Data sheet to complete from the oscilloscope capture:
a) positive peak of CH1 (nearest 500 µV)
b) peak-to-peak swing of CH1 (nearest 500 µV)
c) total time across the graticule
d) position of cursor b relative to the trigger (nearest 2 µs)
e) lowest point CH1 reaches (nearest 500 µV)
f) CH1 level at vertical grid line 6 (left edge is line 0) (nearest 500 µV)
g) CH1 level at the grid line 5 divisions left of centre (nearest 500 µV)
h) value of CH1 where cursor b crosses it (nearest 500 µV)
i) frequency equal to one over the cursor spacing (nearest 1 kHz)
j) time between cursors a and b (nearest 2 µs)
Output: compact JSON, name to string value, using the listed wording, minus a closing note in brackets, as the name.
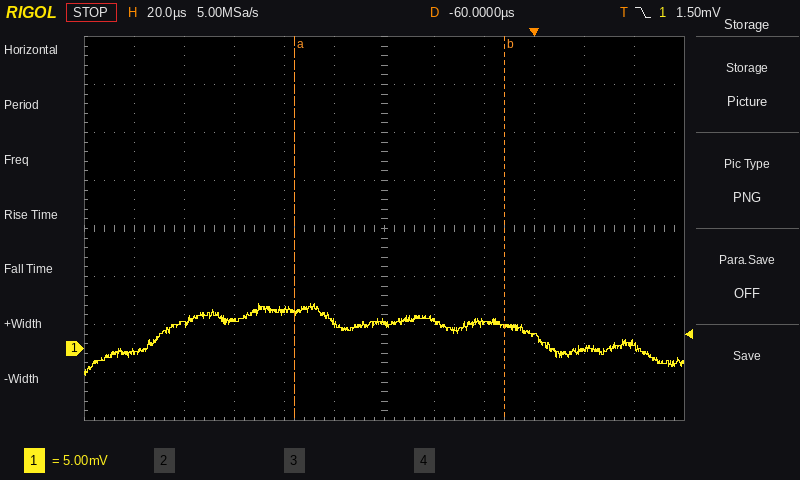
{"positive peak of CH1": "4.5 mV", "peak-to-peak swing of CH1": "7.5 mV", "total time across the graticule": "240 µs", "position of cursor b relative to the trigger": "-12 µs", "lowest point CH1 reaches": "-3.0 mV", "CH1 level at vertical grid line 6 (left edge is line 0)": "2.5 mV", "CH1 level at the grid line 5 divisions left of centre": "-500 µV", "value of CH1 where cursor b crosses it": "2.5 mV", "frequency equal to one over the cursor spacing": "12 kHz", "time between cursors a and b": "84 µs"}
